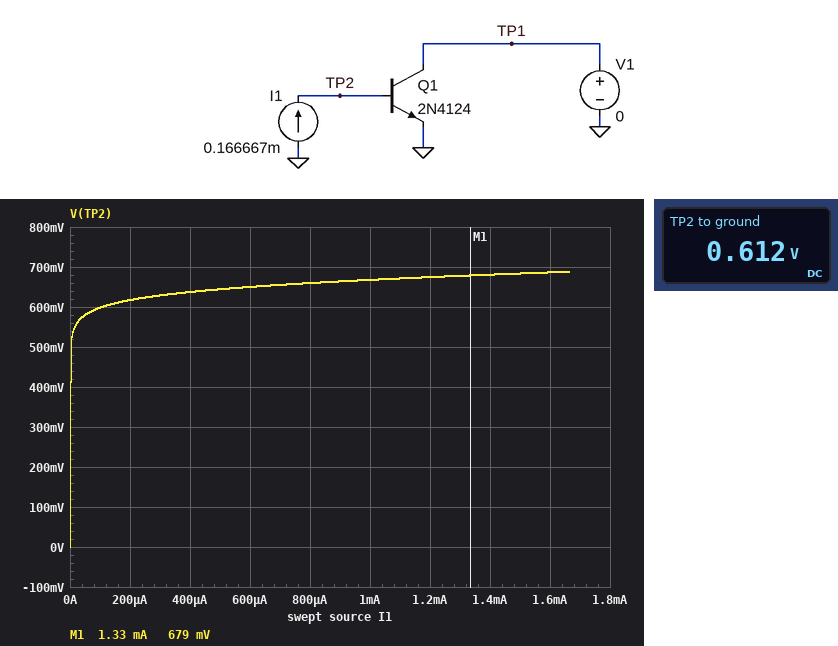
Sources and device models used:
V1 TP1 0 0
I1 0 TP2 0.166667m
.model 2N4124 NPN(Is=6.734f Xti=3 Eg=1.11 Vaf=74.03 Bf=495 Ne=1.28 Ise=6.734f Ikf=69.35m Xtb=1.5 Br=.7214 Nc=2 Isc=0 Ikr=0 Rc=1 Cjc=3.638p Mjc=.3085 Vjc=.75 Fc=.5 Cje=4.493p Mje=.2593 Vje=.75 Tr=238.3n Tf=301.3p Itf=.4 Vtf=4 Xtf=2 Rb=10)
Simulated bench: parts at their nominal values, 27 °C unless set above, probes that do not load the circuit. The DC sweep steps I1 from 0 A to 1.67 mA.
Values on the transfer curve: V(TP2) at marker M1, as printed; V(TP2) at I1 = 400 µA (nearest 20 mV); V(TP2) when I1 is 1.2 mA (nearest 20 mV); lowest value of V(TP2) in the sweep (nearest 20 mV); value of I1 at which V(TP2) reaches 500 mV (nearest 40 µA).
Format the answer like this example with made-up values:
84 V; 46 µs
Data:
679 mV; 640 mV; 680 mV; 0 V; 0 A
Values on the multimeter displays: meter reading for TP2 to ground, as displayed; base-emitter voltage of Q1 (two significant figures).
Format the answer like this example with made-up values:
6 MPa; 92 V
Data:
0.612 V; 610 mV
